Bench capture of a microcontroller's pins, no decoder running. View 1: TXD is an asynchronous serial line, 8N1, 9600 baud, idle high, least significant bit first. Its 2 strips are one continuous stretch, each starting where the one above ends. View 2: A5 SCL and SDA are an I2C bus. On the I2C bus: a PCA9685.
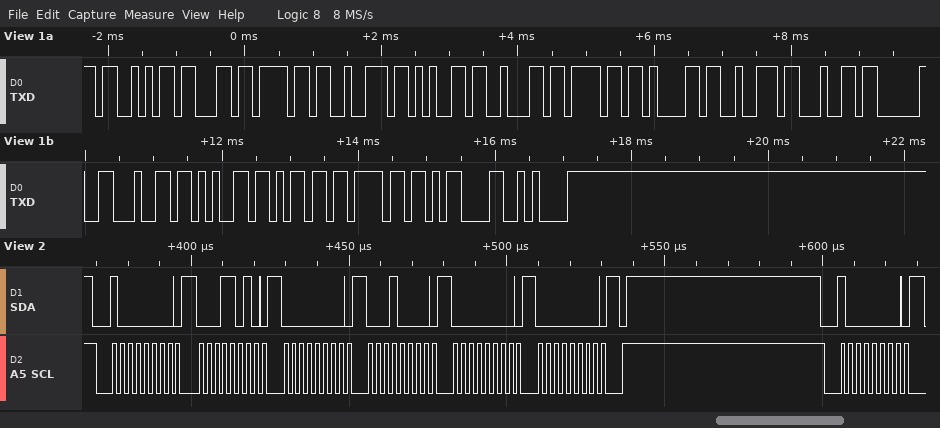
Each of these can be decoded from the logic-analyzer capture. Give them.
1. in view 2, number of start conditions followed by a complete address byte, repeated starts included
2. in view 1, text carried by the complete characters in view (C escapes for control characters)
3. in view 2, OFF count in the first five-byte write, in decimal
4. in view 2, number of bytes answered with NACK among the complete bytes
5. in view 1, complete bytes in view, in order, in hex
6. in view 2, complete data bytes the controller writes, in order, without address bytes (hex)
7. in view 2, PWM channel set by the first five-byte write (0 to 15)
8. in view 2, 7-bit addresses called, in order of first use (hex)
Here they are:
2
"Scoreboard demo\r\n"
0
0
0x53 0x63 0x6F 0x72 0x65 0x62 0x6F 0x61 0x72 0x64 0x20 0x64 0x65 0x6D 0x6F 0x0D 0x0A
1A 00 10 00 00
5
0x40
